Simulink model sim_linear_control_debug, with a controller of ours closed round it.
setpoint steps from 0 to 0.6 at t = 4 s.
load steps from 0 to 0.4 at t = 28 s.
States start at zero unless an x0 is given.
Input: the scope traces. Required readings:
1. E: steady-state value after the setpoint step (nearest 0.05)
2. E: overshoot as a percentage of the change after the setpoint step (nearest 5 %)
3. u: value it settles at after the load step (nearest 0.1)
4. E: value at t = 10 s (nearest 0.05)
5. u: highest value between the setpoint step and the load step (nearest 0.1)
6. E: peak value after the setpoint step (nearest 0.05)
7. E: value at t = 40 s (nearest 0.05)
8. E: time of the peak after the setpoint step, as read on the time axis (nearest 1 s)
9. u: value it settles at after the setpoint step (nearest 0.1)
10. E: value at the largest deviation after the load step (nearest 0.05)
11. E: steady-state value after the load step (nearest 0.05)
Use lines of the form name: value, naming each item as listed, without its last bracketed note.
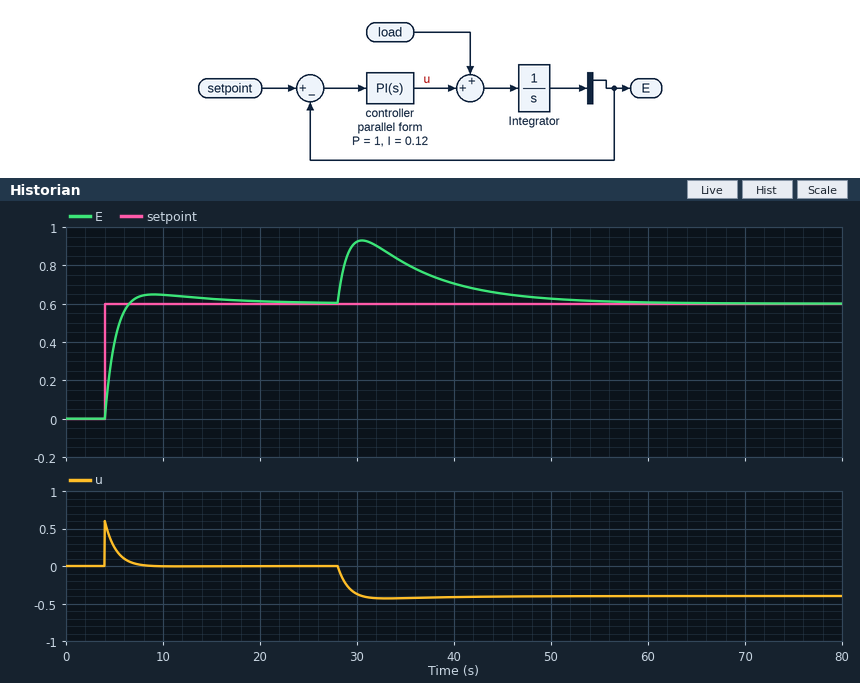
E: steady-state value after the setpoint step: 0.60
E: overshoot as a percentage of the change after the setpoint step: 10 %
u: value it settles at after the load step: -0.4
E: value at t = 10 s: 0.65
u: highest value between the setpoint step and the load step: 0.6
E: peak value after the setpoint step: 0.65
E: value at t = 40 s: 0.70
E: time of the peak after the setpoint step, as read on the time axis: 9 s
u: value it settles at after the setpoint step: 0.0
E: value at the largest deviation after the load step: 0.95
E: steady-state value after the load step: 0.60
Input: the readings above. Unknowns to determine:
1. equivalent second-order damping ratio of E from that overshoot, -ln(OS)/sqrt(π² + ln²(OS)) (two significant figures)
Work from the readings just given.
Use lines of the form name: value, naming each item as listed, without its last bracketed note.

equivalent second-order damping ratio of E from that overshoot, -ln(OS)/sqrt(π² + ln²(OS)): 0.59
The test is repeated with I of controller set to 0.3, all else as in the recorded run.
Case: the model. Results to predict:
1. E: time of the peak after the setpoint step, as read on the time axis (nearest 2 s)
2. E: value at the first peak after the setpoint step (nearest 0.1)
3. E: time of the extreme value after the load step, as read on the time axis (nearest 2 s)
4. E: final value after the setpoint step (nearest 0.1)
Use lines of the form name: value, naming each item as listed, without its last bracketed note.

E: time of the peak after the setpoint step, as read on the time axis: 8 s
E: value at the first peak after the setpoint step: 0.7
E: time of the extreme value after the load step, as read on the time axis: 30 s
E: final value after the setpoint step: 0.6
